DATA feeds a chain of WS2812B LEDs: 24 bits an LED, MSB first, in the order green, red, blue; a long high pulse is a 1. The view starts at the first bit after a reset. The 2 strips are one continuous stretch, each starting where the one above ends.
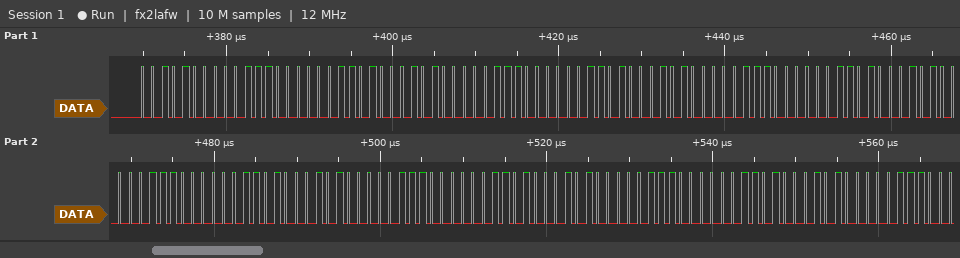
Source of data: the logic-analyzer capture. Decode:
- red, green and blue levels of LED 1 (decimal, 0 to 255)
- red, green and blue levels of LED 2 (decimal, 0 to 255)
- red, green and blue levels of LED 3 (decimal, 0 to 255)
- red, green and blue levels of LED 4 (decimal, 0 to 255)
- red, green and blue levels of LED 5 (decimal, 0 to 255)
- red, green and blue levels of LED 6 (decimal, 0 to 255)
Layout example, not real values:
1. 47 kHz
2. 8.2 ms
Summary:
1. 56, 40, 26
2. 56, 40, 26
3. 56, 40, 26
4. 56, 40, 26
5. 56, 40, 26
6. 56, 40, 26
